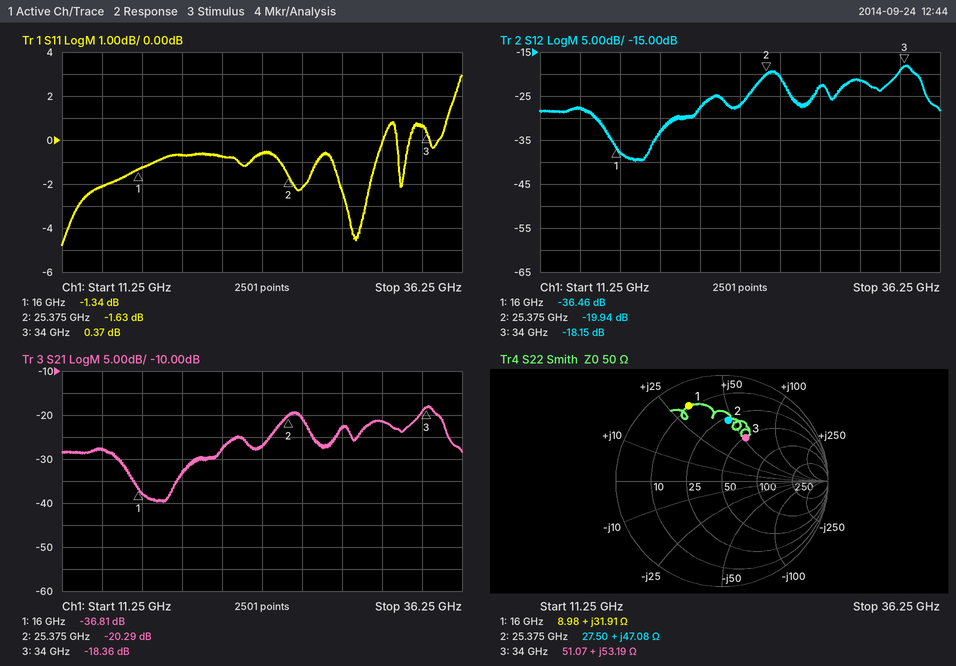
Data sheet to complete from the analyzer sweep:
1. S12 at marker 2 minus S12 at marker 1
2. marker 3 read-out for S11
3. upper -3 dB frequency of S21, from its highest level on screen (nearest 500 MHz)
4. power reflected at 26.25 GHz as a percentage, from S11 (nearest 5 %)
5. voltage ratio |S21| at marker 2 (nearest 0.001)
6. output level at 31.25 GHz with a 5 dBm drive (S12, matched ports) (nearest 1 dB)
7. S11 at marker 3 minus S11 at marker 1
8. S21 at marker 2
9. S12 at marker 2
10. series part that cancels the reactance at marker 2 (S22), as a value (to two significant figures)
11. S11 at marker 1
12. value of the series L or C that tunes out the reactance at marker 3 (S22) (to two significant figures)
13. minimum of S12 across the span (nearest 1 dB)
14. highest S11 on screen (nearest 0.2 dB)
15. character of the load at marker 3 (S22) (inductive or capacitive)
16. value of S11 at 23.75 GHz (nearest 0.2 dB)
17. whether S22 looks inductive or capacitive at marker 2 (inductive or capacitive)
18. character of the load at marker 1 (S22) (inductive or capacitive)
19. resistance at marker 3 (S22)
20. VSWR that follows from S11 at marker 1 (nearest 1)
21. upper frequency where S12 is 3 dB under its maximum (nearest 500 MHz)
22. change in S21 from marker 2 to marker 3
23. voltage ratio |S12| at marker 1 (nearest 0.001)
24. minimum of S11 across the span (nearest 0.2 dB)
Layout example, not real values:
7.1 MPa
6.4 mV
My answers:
16.52 dB
0.37 dB
35.0 GHz
60 %
0.097
-16 dBm
1.71 dB
-20.29 dB
-19.94 dB
130 fF
-1.34 dB
88 fF
-40 dB
3.0 dB
inductive
-0.6 dB
inductive
inductive
51.07 Ω
13
35.0 GHz
1.93 dB
0.015
-4.8 dB
